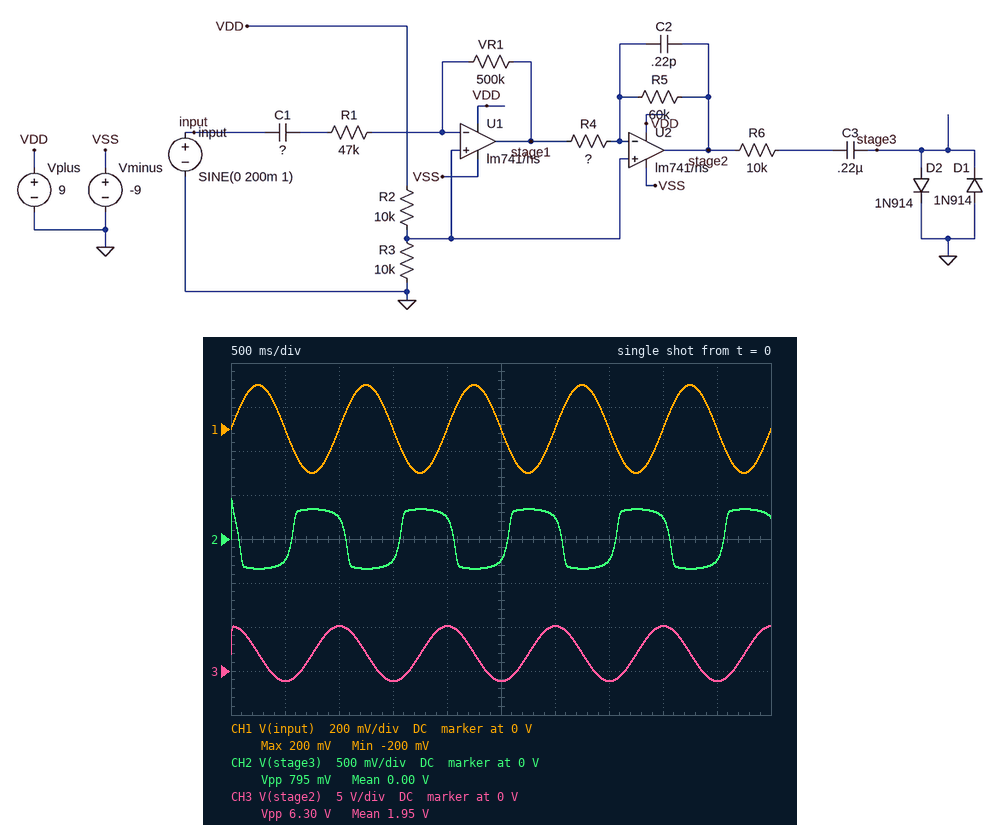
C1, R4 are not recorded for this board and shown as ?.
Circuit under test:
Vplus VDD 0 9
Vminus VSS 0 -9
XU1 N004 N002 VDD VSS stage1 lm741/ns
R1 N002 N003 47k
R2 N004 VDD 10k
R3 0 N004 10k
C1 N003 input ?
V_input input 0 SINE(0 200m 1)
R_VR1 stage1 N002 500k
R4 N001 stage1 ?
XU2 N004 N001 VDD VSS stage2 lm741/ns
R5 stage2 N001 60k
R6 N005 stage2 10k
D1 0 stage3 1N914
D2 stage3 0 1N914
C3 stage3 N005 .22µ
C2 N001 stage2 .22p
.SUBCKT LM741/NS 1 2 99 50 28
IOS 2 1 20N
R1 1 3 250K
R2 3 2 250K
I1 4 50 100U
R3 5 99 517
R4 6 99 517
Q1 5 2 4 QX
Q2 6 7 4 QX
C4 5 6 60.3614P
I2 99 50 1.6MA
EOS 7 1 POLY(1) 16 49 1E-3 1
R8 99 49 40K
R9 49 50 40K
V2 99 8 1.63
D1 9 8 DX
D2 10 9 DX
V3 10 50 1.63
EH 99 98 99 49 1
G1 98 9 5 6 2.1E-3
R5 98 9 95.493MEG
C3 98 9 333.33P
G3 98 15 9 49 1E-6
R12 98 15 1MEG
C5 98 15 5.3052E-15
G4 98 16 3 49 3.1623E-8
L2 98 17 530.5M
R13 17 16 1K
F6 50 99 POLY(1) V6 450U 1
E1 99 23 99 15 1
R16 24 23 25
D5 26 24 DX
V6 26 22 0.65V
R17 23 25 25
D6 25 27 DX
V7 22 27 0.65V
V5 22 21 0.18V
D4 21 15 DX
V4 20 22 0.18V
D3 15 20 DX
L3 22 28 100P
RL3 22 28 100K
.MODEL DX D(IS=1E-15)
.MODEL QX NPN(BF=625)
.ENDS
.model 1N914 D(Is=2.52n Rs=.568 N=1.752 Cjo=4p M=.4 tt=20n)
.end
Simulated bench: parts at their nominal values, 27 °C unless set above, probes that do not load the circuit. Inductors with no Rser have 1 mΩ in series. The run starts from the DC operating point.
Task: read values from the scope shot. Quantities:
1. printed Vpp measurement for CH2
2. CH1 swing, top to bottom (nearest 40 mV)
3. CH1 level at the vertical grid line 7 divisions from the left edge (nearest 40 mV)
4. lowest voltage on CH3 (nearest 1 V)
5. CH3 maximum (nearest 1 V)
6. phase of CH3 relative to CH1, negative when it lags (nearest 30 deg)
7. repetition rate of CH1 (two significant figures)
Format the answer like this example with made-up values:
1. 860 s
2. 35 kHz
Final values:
1. 795 mV
2. 400 mV
3. 0 V
4. -1 V
5. 5 V
6. 90 deg
7. 1.0 Hz
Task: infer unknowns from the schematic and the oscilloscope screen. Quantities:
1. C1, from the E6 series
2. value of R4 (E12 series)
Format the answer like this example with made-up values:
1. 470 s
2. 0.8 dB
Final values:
1. 100 nF
2. 1.2 kΩ
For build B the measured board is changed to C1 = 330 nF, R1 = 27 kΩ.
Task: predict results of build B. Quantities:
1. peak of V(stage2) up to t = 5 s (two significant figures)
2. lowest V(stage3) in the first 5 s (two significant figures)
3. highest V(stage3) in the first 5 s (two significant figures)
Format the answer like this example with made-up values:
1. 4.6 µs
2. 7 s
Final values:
1. 8.0 V
2. -390 mV
3. 500 mV
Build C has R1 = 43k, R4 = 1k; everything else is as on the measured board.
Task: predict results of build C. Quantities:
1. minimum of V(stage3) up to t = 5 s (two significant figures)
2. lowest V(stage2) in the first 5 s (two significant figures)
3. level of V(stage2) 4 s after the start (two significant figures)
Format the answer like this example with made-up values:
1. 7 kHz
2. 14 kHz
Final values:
1. -350 mV
2. -2.3 V
3. 5.2 V
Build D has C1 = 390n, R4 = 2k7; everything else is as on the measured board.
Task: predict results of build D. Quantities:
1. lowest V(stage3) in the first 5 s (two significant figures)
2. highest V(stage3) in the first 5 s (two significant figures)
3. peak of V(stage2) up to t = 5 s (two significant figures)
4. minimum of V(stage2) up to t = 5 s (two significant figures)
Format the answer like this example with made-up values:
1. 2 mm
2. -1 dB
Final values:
1. -360 mV
2. 440 mV
3. 8.0 V
4. -2.0 V
